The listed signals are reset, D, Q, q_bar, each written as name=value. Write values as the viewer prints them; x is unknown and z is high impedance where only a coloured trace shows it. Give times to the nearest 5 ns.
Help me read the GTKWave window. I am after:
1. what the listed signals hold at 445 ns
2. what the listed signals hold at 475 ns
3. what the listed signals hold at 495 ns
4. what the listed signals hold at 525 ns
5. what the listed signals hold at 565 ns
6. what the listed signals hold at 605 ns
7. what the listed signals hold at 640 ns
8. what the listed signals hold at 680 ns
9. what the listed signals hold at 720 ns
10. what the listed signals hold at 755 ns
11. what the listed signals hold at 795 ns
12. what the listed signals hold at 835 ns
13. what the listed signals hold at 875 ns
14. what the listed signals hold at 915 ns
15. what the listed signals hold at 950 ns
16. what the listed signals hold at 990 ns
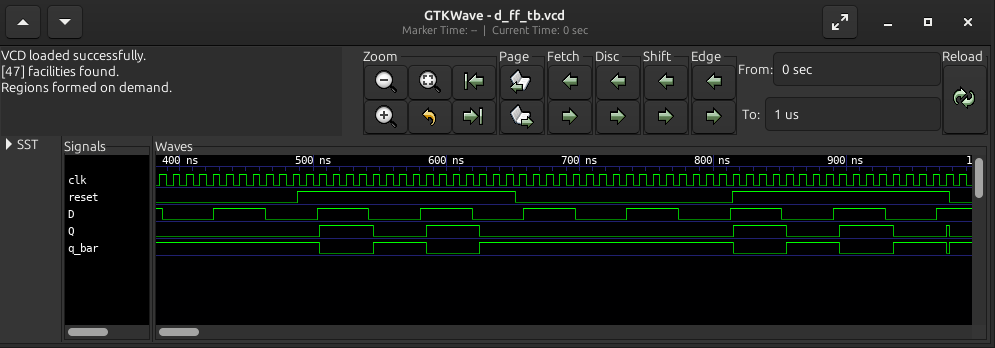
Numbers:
reset=0, D=1, Q=0, q_bar=1
reset=0, D=0, Q=0, q_bar=1
reset=1, D=0, Q=0, q_bar=1
reset=1, D=1, Q=1, q_bar=0
reset=1, D=0, Q=0, q_bar=1
reset=1, D=1, Q=1, q_bar=0
reset=1, D=0, Q=0, q_bar=1
reset=0, D=1, Q=0, q_bar=1
reset=0, D=0, Q=0, q_bar=1
reset=0, D=1, Q=0, q_bar=1
reset=0, D=0, Q=0, q_bar=1
reset=1, D=1, Q=1, q_bar=0
reset=1, D=0, Q=0, q_bar=1
reset=1, D=1, Q=1, q_bar=0
reset=1, D=0, Q=0, q_bar=1
reset=0, D=1, Q=0, q_bar=1
